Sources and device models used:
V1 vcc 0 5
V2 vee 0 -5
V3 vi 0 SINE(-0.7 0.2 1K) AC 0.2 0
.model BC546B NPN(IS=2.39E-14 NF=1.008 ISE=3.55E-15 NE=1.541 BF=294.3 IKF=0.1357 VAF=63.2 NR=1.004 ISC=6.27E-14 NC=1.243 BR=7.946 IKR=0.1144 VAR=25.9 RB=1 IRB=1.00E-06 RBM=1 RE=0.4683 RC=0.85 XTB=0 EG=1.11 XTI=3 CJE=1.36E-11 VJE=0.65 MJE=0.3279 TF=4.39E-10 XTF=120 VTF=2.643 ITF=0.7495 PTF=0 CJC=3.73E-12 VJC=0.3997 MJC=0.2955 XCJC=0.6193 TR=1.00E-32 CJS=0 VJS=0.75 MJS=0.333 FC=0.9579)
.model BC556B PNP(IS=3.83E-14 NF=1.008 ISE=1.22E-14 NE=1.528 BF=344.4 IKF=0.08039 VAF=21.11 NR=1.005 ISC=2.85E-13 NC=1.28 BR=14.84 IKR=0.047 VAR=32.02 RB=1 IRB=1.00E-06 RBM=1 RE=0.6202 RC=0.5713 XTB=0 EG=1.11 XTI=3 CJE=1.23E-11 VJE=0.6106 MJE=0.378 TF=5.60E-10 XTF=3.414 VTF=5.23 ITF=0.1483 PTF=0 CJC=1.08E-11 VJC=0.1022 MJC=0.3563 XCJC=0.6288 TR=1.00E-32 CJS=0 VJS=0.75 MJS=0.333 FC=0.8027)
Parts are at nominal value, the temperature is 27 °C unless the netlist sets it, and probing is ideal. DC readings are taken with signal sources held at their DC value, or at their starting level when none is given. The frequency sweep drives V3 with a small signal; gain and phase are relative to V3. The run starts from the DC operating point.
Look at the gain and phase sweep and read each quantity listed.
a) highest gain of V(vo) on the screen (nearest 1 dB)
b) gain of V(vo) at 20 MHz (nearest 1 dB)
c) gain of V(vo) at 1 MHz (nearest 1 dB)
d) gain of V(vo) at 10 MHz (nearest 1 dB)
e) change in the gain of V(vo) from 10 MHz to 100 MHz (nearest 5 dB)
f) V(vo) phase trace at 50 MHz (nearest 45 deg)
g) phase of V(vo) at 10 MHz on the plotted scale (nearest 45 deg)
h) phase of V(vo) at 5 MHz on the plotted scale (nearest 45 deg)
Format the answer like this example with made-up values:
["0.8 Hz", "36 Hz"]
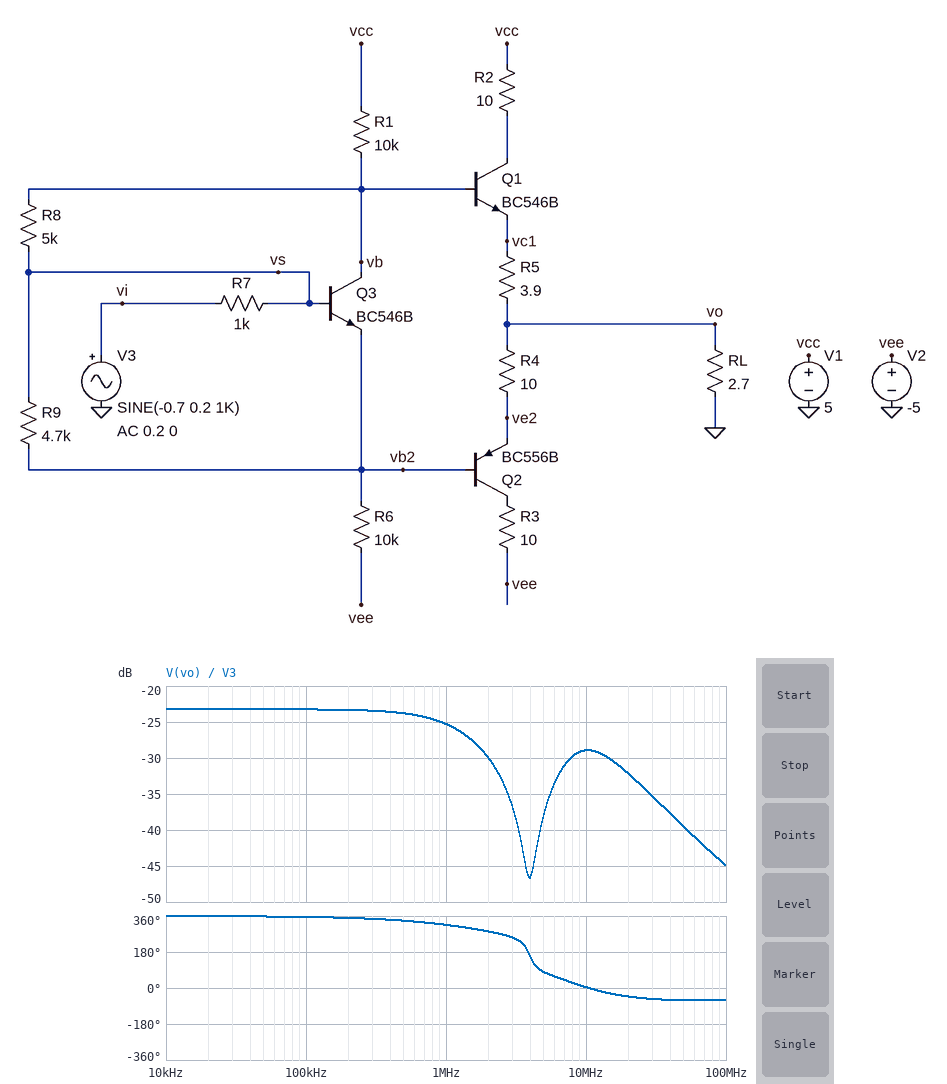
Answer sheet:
["-23 dB", "-32 dB", "-25 dB", "-29 dB", "-15 dB", "-45 deg", "0 deg", "90 deg"]
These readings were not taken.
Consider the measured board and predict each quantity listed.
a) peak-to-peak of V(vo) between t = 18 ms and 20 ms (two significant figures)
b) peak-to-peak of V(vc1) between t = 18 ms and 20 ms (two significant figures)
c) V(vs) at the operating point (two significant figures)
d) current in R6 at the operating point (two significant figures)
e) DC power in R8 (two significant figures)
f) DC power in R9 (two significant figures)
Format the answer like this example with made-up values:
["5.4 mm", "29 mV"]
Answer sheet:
["28 mV", "20 mV", "-570 mV", "380 µA", "320 µW", "73 µW"]
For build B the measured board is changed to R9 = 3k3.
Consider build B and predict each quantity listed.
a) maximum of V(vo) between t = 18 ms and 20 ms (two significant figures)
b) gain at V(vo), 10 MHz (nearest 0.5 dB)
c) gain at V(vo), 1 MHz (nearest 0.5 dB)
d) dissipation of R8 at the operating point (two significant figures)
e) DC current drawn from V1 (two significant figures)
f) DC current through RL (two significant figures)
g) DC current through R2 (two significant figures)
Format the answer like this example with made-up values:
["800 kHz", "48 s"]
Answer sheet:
["-31 mV", "-29.5 dB", "-25.0 dB", "370 µW", "21 mA", "17 mA", "20 mA"]
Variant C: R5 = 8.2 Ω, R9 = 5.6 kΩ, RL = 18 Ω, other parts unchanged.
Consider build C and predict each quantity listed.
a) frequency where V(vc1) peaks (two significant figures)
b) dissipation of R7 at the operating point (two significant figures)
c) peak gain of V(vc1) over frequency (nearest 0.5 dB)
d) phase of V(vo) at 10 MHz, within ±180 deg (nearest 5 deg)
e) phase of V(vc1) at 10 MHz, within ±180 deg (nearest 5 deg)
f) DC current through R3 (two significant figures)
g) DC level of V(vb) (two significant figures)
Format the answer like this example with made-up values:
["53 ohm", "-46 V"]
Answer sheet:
["9.9 MHz", "12 µW", "-11.5 dB", "-15 deg", "75 deg", "21 mA", "500 mV"]
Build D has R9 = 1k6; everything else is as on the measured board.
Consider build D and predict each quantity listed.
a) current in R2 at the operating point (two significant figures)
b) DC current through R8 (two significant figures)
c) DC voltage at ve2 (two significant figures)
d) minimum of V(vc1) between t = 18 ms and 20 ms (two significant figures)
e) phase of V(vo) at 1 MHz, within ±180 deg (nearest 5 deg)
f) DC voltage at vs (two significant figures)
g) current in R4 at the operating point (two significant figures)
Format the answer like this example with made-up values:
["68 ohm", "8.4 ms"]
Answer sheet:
["29 mA", "300 µA", "-360 mV", "60 mV", "-25 deg", "-670 mV", "34 mA"]
